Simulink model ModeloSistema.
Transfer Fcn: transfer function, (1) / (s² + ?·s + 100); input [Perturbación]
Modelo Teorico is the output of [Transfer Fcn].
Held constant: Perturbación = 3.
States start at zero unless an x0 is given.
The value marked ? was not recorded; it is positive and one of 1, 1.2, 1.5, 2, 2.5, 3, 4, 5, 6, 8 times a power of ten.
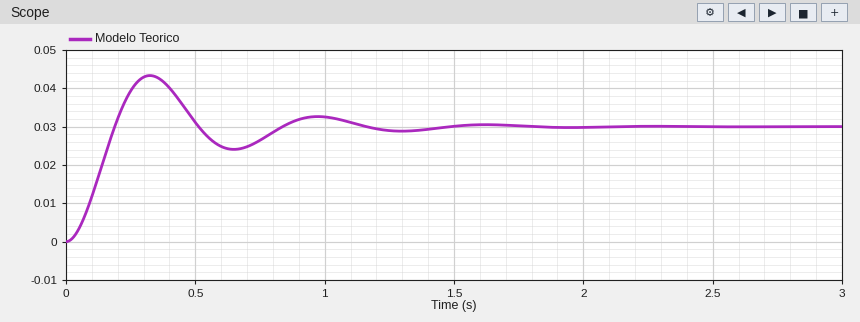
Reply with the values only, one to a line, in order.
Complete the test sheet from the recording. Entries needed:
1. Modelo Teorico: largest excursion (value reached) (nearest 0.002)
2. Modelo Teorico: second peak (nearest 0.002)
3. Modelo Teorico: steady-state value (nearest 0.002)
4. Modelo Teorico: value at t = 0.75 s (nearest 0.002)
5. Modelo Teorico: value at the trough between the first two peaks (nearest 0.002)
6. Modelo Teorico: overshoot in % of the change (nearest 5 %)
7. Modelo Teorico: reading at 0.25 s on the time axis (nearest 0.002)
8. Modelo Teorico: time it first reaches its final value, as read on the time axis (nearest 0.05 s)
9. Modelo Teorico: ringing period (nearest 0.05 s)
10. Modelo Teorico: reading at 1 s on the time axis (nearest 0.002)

0.044
0.032
0.030
0.026
0.024
45 %
0.040
0.20 s
0.65 s
0.032
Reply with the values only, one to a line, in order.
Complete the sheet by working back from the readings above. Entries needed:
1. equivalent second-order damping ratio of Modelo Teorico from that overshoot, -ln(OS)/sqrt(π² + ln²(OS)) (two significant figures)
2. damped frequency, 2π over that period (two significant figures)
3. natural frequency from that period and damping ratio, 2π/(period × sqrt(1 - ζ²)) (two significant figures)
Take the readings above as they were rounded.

0.25
9.7 rad/s
10.0 rad/s
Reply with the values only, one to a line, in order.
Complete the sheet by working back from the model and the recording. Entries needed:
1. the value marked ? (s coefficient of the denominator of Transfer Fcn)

5
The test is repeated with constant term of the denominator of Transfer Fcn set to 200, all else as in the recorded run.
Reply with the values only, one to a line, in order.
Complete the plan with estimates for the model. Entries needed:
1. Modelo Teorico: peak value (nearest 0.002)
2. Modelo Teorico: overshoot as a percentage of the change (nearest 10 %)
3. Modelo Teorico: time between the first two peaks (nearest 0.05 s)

0.024
60 %
0.45 s
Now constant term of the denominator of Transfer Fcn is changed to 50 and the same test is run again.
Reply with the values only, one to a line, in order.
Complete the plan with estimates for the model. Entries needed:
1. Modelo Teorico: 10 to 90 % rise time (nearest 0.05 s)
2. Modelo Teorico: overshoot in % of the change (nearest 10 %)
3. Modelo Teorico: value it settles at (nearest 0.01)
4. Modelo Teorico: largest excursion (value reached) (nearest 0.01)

0.20 s
30 %
0.06
0.08
